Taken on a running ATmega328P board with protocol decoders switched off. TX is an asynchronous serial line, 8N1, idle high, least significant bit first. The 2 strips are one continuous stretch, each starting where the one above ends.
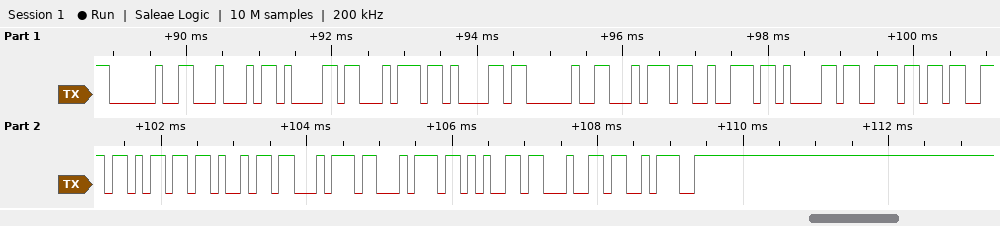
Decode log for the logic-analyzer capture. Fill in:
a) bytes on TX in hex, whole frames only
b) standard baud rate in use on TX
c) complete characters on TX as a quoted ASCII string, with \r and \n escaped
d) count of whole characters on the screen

20 44 61 74 61 20 74 72 61 6E 73 6D 69 74 74 65 64 3A
9600 baud
" Data transmitted:"
18
